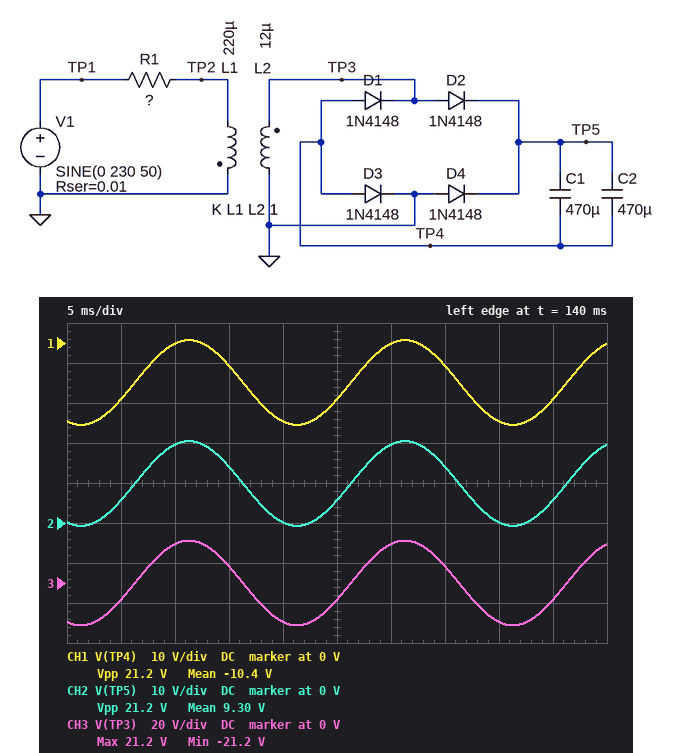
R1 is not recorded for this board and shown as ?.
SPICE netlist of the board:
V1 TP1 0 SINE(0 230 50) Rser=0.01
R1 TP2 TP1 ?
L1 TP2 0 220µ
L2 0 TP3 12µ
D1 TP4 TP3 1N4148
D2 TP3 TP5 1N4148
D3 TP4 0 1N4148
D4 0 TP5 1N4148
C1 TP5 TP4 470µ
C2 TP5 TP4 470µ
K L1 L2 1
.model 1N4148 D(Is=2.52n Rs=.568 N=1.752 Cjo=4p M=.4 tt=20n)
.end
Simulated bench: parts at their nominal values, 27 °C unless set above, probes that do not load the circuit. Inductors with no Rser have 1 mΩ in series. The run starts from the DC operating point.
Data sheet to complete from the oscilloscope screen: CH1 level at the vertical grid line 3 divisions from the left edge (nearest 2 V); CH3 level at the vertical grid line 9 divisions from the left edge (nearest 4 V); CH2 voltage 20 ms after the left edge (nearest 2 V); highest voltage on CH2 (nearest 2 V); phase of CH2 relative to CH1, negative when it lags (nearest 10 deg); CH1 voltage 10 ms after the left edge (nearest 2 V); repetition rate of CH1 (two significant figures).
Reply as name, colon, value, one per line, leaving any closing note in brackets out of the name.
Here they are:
CH1 level at the vertical grid line 3 divisions from the left edge: -6 V
CH3 level at the vertical grid line 9 divisions from the left edge: -8 V
CH2 voltage 20 ms after the left edge: 0 V
highest voltage on CH2: 20 V
phase of CH2 relative to CH1, negative when it lags: 0 deg
CH1 voltage 10 ms after the left edge: 0 V
repetition rate of CH1: 50 Hz
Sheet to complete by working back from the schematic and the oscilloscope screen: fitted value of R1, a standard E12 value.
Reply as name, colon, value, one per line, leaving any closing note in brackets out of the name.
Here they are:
fitted value of R1, a standard E12 value: 0.15 Ω
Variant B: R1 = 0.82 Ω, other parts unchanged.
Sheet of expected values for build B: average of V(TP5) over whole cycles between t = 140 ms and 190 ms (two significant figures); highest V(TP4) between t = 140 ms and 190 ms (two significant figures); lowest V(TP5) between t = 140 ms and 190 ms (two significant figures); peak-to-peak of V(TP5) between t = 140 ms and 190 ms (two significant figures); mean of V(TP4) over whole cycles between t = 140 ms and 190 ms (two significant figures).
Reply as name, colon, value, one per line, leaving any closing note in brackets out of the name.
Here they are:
average of V(TP5) over whole cycles between t = 140 ms and 190 ms: 1.6 V
highest V(TP4) between t = 140 ms and 190 ms: 670 mV
lowest V(TP5) between t = 140 ms and 190 ms: -670 mV
peak-to-peak of V(TP5) between t = 140 ms and 190 ms: 4.5 V
mean of V(TP4) over whole cycles between t = 140 ms and 190 ms: -1.6 V
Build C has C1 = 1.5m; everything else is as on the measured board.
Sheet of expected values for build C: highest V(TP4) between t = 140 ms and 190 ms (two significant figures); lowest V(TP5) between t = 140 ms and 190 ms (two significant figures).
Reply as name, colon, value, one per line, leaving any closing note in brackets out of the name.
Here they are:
highest V(TP4) between t = 140 ms and 190 ms: 790 mV
lowest V(TP5) between t = 140 ms and 190 ms: -800 mV
